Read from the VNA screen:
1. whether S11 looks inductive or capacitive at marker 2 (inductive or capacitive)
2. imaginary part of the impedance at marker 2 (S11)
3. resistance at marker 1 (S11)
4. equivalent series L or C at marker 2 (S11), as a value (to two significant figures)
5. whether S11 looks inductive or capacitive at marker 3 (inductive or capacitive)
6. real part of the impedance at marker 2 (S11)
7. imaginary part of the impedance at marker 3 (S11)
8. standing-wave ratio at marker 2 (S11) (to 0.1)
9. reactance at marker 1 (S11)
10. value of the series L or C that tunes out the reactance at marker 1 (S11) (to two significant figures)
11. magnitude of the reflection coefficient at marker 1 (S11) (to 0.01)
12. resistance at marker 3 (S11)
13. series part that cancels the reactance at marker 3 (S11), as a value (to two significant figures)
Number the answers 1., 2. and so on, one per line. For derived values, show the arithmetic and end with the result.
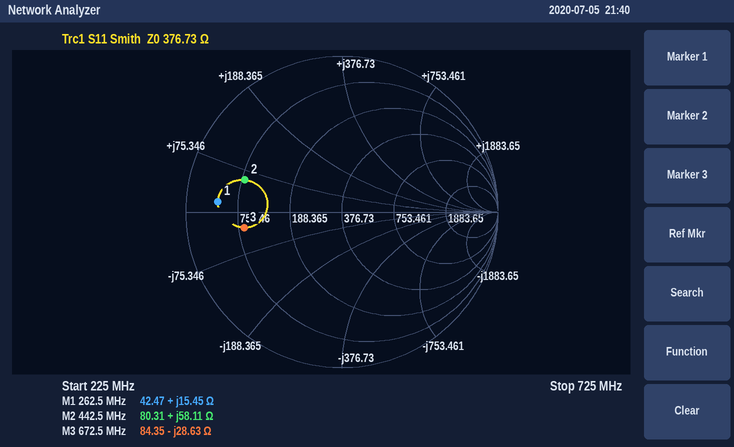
1. inductive
2. +58.11 Ω
3. 42.47 Ω
4. L = 58.11 Ω/(2π × 442.5 MHz) ≈ 21 nH
5. capacitive
6. 80.31 Ω
7. -28.63 Ω
8. 4.8
9. +15.45 Ω
10. C = 1/(2π × 262.5 MHz × 15.45 Ω) ≈ 39 pF
11. 0.80
12. 84.35 Ω
13. L = 28.63 Ω/(2π × 672.5 MHz) ≈ 6.8 nH
